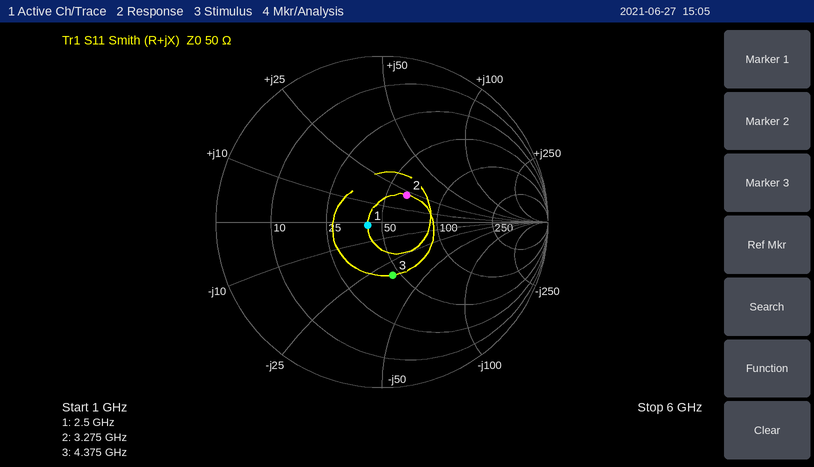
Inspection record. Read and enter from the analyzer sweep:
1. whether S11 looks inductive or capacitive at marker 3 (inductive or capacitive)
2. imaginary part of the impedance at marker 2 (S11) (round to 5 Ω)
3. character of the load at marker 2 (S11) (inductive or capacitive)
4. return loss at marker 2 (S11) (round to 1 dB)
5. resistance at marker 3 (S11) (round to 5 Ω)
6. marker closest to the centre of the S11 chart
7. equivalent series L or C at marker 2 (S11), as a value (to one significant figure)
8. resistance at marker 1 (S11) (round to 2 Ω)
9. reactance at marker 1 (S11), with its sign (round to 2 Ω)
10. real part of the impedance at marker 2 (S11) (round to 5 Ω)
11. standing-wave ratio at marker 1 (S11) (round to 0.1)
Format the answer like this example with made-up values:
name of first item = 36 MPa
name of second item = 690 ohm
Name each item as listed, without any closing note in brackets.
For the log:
whether S11 looks inductive or capacitive at marker 3 = capacitive
imaginary part of the impedance at marker 2 (S11) = +20 Ω
character of the load at marker 2 (S11) = inductive
return loss at marker 2 (S11) = 13 dB
resistance at marker 3 (S11) = 45 Ω
marker closest to the centre of the S11 chart = marker 1
equivalent series L or C at marker 2 (S11), as a value = 1 nH
resistance at marker 1 (S11) = 42 Ω
reactance at marker 1 (S11), with its sign = -2 Ω
real part of the impedance at marker 2 (S11) = 65 Ω
standing-wave ratio at marker 1 (S11) = 1.2
